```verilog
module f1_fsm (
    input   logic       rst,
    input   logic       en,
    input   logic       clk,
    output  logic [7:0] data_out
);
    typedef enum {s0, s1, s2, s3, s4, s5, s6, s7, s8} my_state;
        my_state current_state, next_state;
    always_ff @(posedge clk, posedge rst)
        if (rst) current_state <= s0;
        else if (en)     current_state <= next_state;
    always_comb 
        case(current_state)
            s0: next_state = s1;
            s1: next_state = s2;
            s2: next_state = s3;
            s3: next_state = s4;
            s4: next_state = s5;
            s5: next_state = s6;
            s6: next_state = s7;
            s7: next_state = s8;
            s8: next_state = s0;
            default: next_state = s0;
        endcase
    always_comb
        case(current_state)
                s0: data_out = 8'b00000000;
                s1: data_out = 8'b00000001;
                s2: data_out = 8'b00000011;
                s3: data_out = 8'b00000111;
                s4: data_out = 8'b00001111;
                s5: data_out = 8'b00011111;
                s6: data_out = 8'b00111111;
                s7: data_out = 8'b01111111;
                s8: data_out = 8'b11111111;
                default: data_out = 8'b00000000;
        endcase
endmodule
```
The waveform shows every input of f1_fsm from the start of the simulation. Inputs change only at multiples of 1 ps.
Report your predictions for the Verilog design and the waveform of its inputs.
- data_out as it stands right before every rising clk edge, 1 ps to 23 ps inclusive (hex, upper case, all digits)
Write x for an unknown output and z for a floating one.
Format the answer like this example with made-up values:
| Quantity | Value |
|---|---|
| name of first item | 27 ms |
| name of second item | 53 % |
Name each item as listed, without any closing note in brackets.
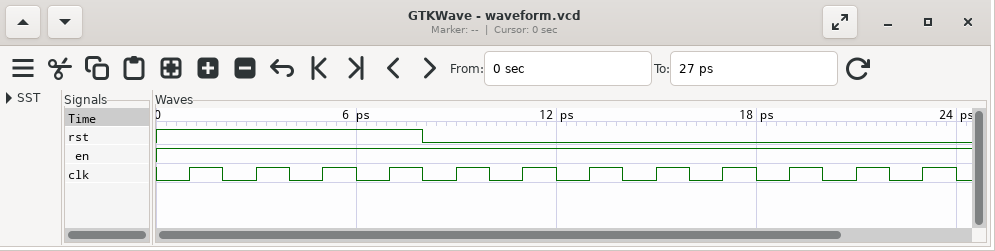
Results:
| Quantity | Value |
|---|---|
| data_out as it stands right before every rising clk edge, 1 ps to 23 ps inclusive | 00, 00, 00, 00, 00, 01, 03, 07, 0F, 1F, 3F, 7F |
